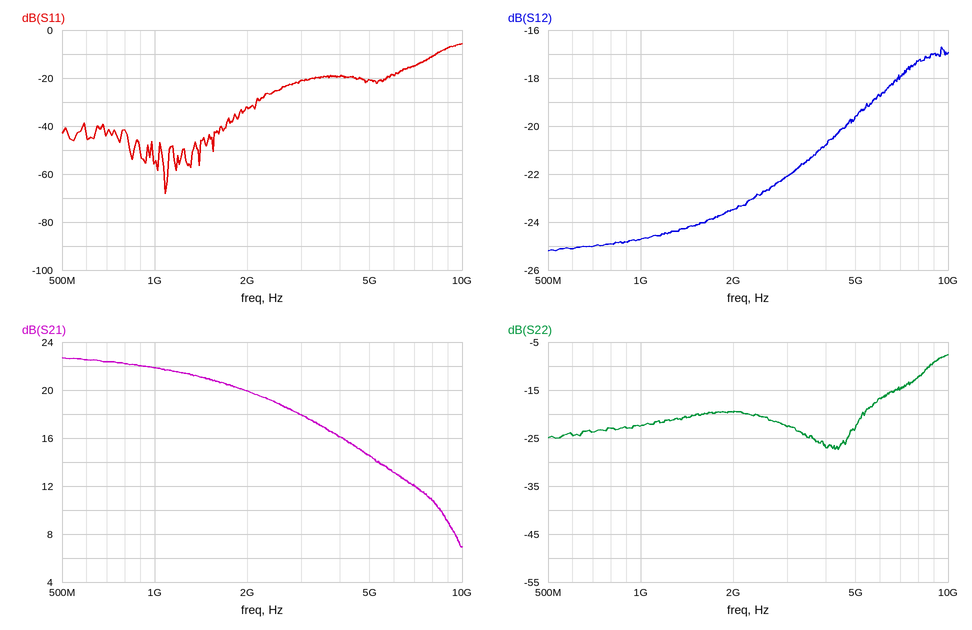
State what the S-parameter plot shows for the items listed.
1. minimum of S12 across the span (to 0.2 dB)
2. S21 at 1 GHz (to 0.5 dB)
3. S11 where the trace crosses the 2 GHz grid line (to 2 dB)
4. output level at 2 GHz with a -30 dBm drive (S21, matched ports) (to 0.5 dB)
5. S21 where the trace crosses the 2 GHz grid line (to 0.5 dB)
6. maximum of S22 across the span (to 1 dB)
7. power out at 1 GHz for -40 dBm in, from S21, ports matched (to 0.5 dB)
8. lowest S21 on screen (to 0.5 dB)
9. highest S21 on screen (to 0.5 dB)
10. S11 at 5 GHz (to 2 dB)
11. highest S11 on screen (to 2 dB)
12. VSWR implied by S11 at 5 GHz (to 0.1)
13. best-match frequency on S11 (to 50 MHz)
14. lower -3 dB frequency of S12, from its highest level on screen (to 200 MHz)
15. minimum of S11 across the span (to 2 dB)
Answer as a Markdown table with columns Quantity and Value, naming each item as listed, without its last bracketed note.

| Quantity | Value |
|---|---|
| minimum of S12 across the span | -25.2 dB |
| S21 at 1 GHz | 22.0 dB |
| S11 where the trace crosses the 2 GHz grid line | -32 dB |
| output level at 2 GHz with a -30 dBm drive (S21, matched ports) | -10.0 dBm |
| S21 where the trace crosses the 2 GHz grid line | 20.0 dB |
| maximum of S22 across the span | -8 dB |
| power out at 1 GHz for -40 dBm in, from S21, ports matched | -18.0 dBm |
| lowest S21 on screen | 7.0 dB |
| highest S21 on screen | 22.5 dB |
| S11 at 5 GHz | -20 dB |
| highest S11 on screen | -6 dB |
| VSWR implied by S11 at 5 GHz | 1.2 |
| best-match frequency on S11 | 1.10 GHz |
| lower -3 dB frequency of S12, from its highest level on screen | 5.0 GHz |
| minimum of S11 across the span | -68 dB |
